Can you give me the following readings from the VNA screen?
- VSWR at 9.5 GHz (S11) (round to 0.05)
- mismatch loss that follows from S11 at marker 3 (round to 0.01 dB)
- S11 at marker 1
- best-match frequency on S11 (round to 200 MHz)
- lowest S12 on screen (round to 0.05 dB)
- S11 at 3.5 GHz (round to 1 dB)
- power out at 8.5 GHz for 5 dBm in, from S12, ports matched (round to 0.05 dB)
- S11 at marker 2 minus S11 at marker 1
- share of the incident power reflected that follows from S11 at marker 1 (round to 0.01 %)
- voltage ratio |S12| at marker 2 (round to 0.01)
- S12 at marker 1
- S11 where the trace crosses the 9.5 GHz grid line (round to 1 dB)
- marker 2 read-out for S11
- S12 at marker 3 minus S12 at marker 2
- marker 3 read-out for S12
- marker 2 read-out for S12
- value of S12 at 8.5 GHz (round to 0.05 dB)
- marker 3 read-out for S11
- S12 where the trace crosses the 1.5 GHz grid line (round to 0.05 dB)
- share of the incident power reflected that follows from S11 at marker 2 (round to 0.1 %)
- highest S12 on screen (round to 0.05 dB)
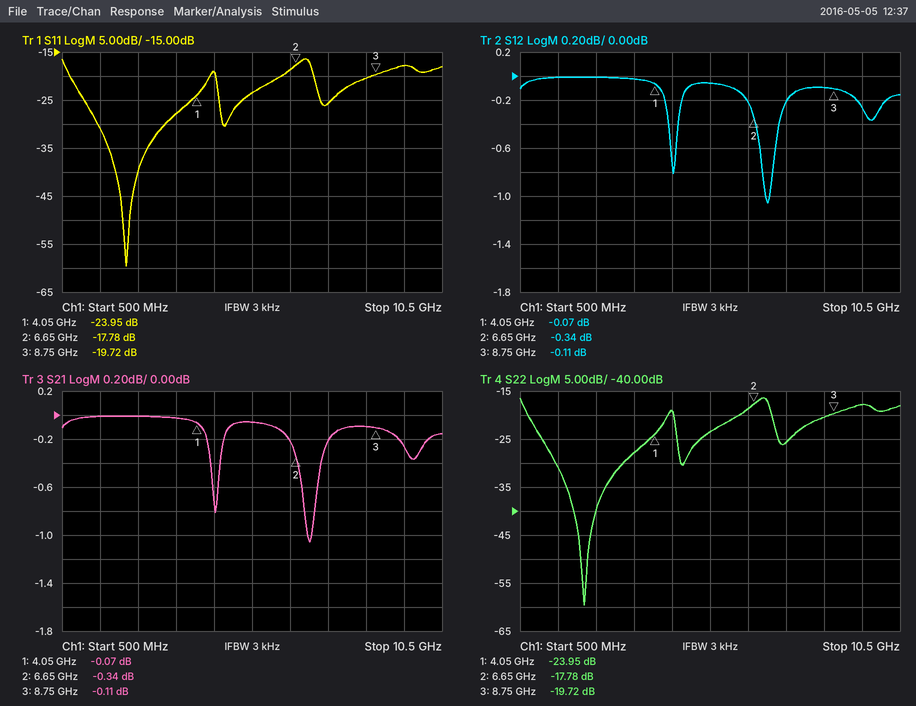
1.30
0.05 dB
-23.95 dB
2.2 GHz
-1.05 dB
-28 dB
4.90 dBm
6.17 dB
0.40 %
0.96
-0.07 dB
-18 dB
-17.78 dB
0.23 dB
-0.11 dB
-0.34 dB
-0.10 dB
-19.72 dB
0.00 dB
1.7 %
0.00 dB
